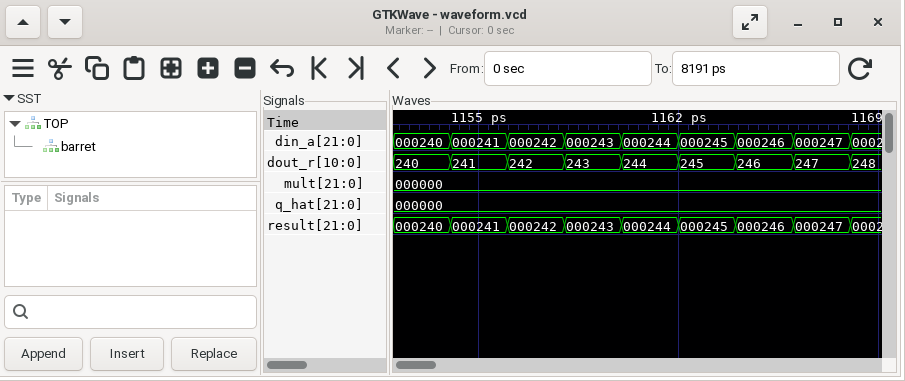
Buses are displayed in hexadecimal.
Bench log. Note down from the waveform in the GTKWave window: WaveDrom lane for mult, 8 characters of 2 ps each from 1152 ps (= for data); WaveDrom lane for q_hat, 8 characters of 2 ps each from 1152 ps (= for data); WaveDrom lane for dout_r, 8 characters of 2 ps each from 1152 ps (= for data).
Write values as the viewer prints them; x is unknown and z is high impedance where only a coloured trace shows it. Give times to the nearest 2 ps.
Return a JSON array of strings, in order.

["{name: 'mult', wave: '=.......', data: '000000'}", "{name: 'q_hat', wave: '=.......', data: '000000'}", "{name: 'dout_r', wave: '========', data: '240 241 242 243 244 245 246 247'}"]
